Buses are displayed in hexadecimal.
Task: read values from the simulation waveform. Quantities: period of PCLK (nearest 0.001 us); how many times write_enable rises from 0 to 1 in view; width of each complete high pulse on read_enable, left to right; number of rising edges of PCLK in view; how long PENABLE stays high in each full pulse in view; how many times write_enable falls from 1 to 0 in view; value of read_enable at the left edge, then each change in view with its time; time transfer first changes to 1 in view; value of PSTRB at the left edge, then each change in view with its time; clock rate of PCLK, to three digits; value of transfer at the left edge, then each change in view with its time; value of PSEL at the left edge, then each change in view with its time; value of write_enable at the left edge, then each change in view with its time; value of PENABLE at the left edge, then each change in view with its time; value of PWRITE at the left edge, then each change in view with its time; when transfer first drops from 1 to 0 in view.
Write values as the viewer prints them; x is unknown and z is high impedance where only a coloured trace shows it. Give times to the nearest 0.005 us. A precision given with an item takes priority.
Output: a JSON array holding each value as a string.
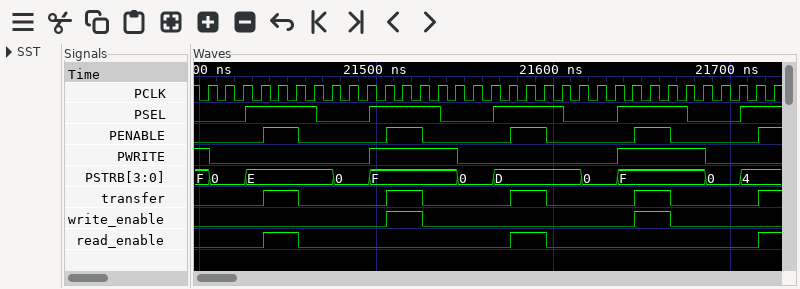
["0.01 us", "2", "0.02 us, 0.02 us", "33", "0.02 us, 0.02 us, 0.02 us, 0.02 us", "2", "0, 1 at 21.435 us, 0 at 21.455 us, 1 at 21.575 us, 0 at 21.595 us, 1 at 21.715 us", "21.435 us", "F, 0 at 21.405 us, E at 21.425 us, 0 at 21.475 us, F at 21.495 us, 0 at 21.545 us, D at 21.565 us, 0 at 21.615 us, F at 21.635 us, 0 at 21.685 us, 4 at 21.705 us", "100 MHz", "0, 1 at 21.435 us, 0 at 21.455 us, 1 at 21.505 us, 0 at 21.525 us, 1 at 21.575 us, 0 at 21.595 us, 1 at 21.645 us, 0 at 21.665 us, 1 at 21.715 us", "0, 1 at 21.425 us, 0 at 21.465 us, 1 at 21.495 us, 0 at 21.535 us, 1 at 21.565 us, 0 at 21.605 us, 1 at 21.635 us, 0 at 21.675 us, 1 at 21.705 us", "0, 1 at 21.505 us, 0 at 21.525 us, 1 at 21.645 us, 0 at 21.665 us", "0, 1 at 21.435 us, 0 at 21.455 us, 1 at 21.505 us, 0 at 21.525 us, 1 at 21.575 us, 0 at 21.595 us, 1 at 21.645 us, 0 at 21.665 us, 1 at 21.715 us", "1, 0 at 21.405 us, 1 at 21.495 us, 0 at 21.545 us, 1 at 21.635 us, 0 at 21.685 us", "21.455 us"]
